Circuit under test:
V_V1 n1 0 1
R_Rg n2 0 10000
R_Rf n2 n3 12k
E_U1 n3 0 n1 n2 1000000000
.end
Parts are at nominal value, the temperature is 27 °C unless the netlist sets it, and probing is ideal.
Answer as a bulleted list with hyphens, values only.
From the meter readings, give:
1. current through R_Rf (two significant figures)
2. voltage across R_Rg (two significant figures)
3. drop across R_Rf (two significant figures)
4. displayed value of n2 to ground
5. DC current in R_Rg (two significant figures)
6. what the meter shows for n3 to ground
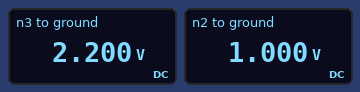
- 100 µA
- 1.0 V
- 1.2 V
- 1.000 V
- 100 µA
- 2.200 V
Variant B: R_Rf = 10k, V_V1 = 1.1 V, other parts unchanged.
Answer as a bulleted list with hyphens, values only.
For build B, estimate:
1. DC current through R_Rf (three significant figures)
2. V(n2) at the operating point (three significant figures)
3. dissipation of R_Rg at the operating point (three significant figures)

- 110 µA
- 1.10 V
- 121 µW
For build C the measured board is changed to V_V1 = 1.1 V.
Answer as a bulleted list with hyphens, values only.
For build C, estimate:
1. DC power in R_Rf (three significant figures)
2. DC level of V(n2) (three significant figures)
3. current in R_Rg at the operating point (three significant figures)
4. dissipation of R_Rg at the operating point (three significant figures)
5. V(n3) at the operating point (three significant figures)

- 145 µW
- 1.10 V
- 110 µA
- 121 µW
- 2.42 V
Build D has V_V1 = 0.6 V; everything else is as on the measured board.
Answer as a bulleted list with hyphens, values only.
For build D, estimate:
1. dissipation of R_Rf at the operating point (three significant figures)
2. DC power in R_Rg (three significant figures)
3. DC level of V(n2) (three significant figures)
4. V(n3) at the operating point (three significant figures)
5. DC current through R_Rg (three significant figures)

- 43.2 µW
- 36.0 µW
- 600 mV
- 1.32 V
- 60.0 µA
